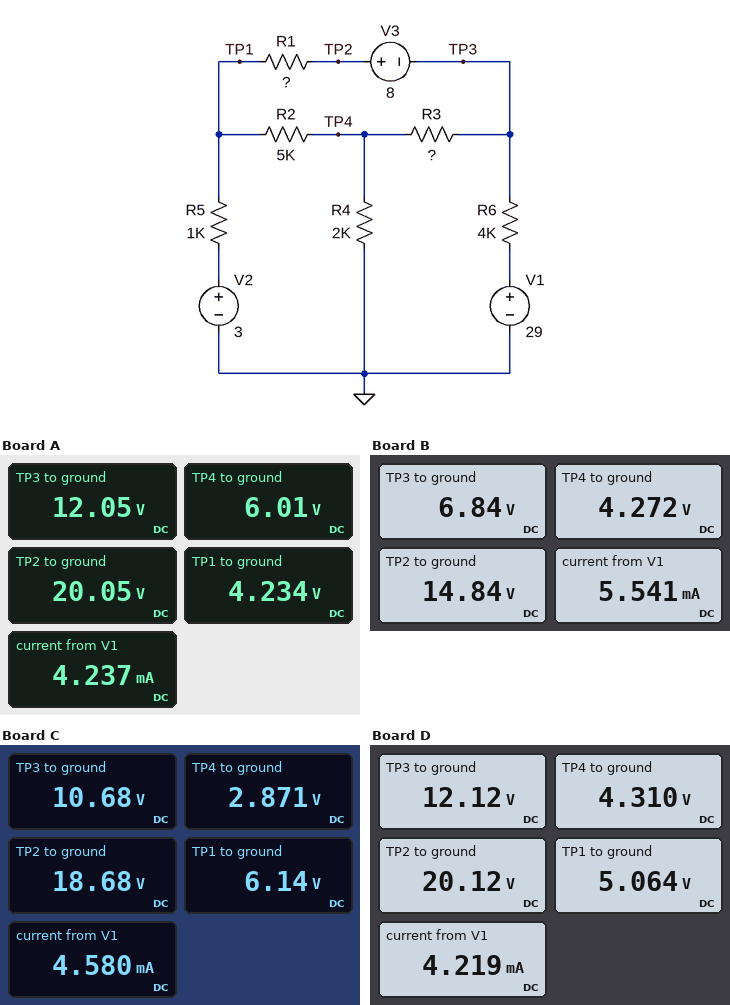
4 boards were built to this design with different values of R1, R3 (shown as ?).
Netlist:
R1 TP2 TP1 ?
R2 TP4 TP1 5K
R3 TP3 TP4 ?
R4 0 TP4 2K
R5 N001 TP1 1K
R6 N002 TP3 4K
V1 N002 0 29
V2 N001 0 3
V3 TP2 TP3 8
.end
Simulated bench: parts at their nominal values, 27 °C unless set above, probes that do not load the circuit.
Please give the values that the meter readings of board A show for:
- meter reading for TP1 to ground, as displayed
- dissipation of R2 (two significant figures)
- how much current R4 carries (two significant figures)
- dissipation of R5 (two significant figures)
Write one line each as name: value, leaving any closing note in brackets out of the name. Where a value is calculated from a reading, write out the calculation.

meter reading for TP1 to ground, as displayed: 4.234 V
dissipation of R2: (6.01 V - 4.234 V)^2 / 5 kΩ = 630 µW
how much current R4 carries: (6.01 V) / 2 kΩ = 3.0 mA
dissipation of R5: (4.234 V - 3 V)^2 / 1 kΩ = 1.5 mW
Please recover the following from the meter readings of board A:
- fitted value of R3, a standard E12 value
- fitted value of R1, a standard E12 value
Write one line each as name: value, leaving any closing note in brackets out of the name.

fitted value of R3, a standard E12 value: 1.8 kΩ
fitted value of R1, a standard E12 value: 18 kΩ
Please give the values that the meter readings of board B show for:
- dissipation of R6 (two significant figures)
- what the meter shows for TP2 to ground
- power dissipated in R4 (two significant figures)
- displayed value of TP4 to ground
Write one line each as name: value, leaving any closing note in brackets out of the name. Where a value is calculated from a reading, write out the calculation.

dissipation of R6: (29 V - 6.84 V)^2 / 4 kΩ = 120 mW
what the meter shows for TP2 to ground: 14.84 V
power dissipated in R4: (4.272 V)^2 / 2 kΩ = 9.1 mW
displayed value of TP4 to ground: 4.272 V
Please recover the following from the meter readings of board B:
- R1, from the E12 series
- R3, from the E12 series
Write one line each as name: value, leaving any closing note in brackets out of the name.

R1, from the E12 series: 2.2 kΩ
R3, from the E12 series: 1.5 kΩ
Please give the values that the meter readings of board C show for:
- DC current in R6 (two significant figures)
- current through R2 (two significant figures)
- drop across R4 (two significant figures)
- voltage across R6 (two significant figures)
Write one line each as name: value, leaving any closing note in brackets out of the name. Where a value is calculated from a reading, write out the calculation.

DC current in R6: (29 V - 10.68 V) / 4 kΩ = 4.6 mA
current through R2: (6.14 V - 2.871 V) / 5 kΩ = 650 µA
drop across R4: 2.871 V = 2.9 V
voltage across R6: 29 V - 10.68 V = 18 V
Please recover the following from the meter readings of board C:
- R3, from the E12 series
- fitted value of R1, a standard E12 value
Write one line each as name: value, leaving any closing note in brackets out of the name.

R3, from the E12 series: 10 kΩ
fitted value of R1, a standard E12 value: 3.3 kΩ
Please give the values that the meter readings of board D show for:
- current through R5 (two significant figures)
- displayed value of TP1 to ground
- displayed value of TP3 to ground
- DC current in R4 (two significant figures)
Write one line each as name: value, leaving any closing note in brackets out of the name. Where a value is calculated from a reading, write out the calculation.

current through R5: (5.064 V - 3 V) / 1 kΩ = 2.1 mA
displayed value of TP1 to ground: 5.064 V
displayed value of TP3 to ground: 12.12 V
DC current in R4: (4.31 V) / 2 kΩ = 2.2 mA
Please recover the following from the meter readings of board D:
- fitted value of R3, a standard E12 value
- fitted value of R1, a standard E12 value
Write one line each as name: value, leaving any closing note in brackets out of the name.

fitted value of R3, a standard E12 value: 3.9 kΩ
fitted value of R1, a standard E12 value: 6.8 kΩ
